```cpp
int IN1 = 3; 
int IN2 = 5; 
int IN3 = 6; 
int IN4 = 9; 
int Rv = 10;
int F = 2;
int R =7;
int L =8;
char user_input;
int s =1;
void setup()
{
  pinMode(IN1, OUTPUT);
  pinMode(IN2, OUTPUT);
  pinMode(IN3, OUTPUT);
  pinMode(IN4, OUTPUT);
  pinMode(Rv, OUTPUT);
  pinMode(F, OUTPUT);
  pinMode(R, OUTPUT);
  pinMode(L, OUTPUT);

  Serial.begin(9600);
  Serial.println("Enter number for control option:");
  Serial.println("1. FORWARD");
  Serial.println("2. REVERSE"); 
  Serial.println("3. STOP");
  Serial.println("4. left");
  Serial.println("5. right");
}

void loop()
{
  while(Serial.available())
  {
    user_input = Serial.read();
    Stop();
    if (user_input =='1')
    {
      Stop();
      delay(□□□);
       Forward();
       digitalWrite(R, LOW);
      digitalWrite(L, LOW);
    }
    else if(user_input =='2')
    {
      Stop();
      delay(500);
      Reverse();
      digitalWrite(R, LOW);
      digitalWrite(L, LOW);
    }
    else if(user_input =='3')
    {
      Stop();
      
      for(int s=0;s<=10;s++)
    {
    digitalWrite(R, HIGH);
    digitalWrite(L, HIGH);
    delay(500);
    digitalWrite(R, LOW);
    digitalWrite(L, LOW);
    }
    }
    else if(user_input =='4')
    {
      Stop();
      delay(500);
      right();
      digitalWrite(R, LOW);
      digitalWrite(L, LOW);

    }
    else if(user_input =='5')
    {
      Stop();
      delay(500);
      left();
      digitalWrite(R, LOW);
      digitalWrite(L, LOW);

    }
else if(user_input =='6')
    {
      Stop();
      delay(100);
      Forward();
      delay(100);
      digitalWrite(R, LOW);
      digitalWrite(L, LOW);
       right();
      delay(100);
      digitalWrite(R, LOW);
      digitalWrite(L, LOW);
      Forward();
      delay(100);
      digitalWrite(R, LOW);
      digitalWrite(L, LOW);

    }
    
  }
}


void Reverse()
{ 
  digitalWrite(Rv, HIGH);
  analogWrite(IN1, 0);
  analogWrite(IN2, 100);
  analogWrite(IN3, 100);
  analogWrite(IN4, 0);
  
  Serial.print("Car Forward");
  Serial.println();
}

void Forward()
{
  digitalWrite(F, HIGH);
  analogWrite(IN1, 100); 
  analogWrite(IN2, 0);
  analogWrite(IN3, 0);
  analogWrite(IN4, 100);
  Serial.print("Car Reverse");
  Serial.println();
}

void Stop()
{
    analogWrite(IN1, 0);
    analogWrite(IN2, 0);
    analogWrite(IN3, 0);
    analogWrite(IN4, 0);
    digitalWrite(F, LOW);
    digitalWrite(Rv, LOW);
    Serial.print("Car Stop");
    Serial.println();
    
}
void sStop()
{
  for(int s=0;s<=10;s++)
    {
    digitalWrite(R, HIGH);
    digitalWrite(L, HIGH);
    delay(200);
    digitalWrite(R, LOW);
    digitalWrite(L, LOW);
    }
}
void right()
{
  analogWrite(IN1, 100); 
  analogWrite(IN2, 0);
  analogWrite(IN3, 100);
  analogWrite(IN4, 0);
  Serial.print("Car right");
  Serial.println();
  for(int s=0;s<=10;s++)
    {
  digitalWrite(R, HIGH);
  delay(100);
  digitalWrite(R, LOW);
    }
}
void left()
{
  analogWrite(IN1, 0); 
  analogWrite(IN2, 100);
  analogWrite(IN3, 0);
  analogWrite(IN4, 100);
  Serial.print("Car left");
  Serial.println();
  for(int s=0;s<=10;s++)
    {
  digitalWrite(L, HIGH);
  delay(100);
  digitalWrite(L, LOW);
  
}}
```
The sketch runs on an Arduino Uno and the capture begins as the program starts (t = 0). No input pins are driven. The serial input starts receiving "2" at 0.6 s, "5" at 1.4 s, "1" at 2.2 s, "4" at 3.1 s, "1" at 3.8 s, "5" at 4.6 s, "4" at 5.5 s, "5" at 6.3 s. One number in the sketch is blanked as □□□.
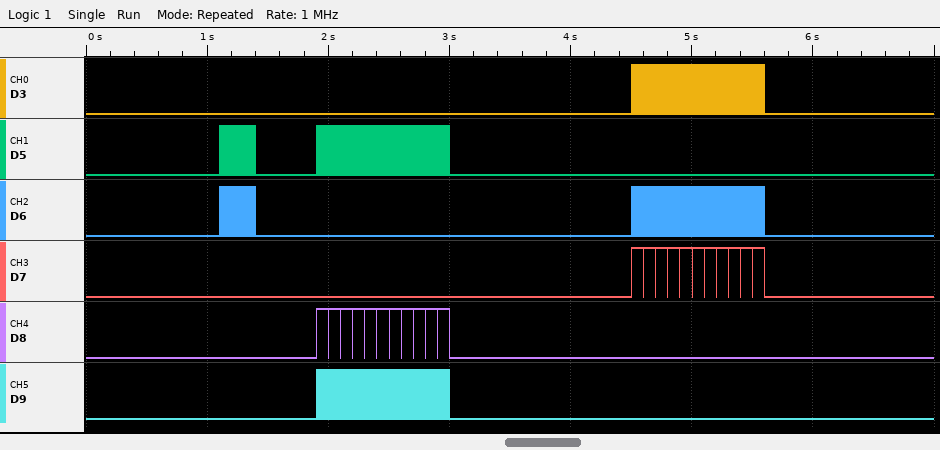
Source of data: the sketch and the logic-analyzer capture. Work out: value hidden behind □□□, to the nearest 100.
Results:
1000
